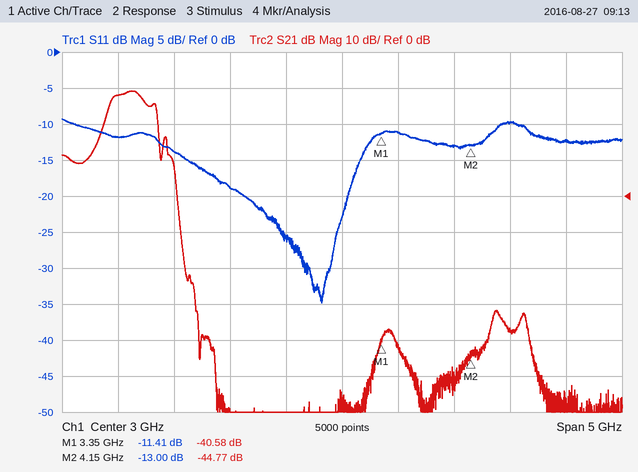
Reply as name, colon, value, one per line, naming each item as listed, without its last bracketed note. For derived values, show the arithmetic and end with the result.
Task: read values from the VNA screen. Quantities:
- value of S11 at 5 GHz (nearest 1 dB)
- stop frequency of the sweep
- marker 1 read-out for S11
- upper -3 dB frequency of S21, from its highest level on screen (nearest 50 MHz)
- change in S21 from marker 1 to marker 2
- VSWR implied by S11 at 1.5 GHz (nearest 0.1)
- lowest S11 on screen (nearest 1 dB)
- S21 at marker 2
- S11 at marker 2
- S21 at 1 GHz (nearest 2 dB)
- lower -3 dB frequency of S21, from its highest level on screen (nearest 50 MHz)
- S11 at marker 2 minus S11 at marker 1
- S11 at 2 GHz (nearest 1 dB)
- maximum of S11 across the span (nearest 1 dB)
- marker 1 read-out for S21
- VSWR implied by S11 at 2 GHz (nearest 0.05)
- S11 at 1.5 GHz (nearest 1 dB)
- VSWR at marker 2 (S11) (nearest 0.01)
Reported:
value of S11 at 5 GHz: -12 dB
stop frequency of the sweep: 5.5 GHz
marker 1 read-out for S11: -11.41 dB
upper -3 dB frequency of S21, from its highest level on screen: 1.25 GHz
change in S21 from marker 1 to marker 2: -44.77 − (-40.58) = -4.19 dB
VSWR implied by S11 at 1.5 GHz: |Γ| = 10^(-14/20) = 0.1995; VSWR = (1 + 0.1995)/(1 − 0.1995) ≈ 1.5
lowest S11 on screen: -35 dB
S21 at marker 2: -44.77 dB
S11 at marker 2: -13.00 dB
S21 at 1 GHz: 28 dB
lower -3 dB frequency of S21, from its highest level on screen: 950 MHz
S11 at marker 2 minus S11 at marker 1: -13 − (-11.41) = -1.59 dB
S11 at 2 GHz: -19 dB
maximum of S11 across the span: -9 dB
marker 1 read-out for S21: -40.58 dB
VSWR implied by S11 at 2 GHz: |Γ| = 10^(-19/20) = 0.1122; VSWR = (1 + 0.1122)/(1 − 0.1122) ≈ 1.25
S11 at 1.5 GHz: -14 dB
VSWR at marker 2 (S11): (1 + 0.2239)/(1 − 0.2239) ≈ 1.58
